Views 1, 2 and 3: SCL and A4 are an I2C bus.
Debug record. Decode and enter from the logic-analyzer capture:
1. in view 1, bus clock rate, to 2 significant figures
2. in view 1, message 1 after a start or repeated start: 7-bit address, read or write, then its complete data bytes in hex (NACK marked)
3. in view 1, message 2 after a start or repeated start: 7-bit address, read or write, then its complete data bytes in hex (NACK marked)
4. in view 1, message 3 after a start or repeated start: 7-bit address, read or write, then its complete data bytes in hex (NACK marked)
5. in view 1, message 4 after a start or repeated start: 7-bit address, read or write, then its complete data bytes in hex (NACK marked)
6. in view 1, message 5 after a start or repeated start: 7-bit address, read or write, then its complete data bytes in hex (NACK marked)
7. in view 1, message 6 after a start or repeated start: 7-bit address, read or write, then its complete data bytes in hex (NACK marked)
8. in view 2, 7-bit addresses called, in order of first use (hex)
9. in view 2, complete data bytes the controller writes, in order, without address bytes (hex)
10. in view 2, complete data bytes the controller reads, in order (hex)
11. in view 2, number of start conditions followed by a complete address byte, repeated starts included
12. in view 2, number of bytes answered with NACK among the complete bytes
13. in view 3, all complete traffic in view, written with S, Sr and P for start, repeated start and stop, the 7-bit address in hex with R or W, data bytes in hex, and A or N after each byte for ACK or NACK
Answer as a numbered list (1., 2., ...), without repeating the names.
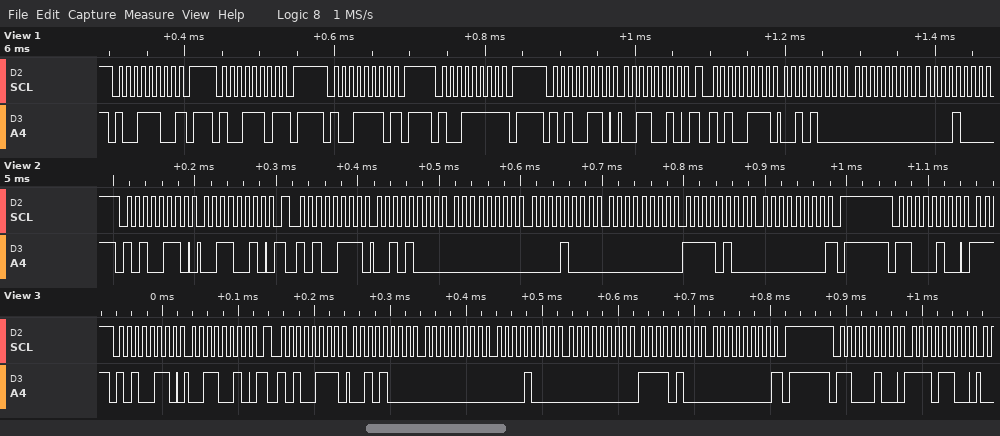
1. 100 kHz
2. 0x4E write NACK
3. 0x4E read NACK
4. 0x4F write NACK
5. 0x4F read NACK
6. 0x53 write: 32
7. 0x53 read: 28 00 08
8. 0x53 0x62
9. 32
10. 28 00 08 00 F4 00
11. 3
12. 1
13. S 53W A 32 A Sr 53R A 28 A 00 A 08 A 00 A F4 A 00 N P S 62W A EC A
